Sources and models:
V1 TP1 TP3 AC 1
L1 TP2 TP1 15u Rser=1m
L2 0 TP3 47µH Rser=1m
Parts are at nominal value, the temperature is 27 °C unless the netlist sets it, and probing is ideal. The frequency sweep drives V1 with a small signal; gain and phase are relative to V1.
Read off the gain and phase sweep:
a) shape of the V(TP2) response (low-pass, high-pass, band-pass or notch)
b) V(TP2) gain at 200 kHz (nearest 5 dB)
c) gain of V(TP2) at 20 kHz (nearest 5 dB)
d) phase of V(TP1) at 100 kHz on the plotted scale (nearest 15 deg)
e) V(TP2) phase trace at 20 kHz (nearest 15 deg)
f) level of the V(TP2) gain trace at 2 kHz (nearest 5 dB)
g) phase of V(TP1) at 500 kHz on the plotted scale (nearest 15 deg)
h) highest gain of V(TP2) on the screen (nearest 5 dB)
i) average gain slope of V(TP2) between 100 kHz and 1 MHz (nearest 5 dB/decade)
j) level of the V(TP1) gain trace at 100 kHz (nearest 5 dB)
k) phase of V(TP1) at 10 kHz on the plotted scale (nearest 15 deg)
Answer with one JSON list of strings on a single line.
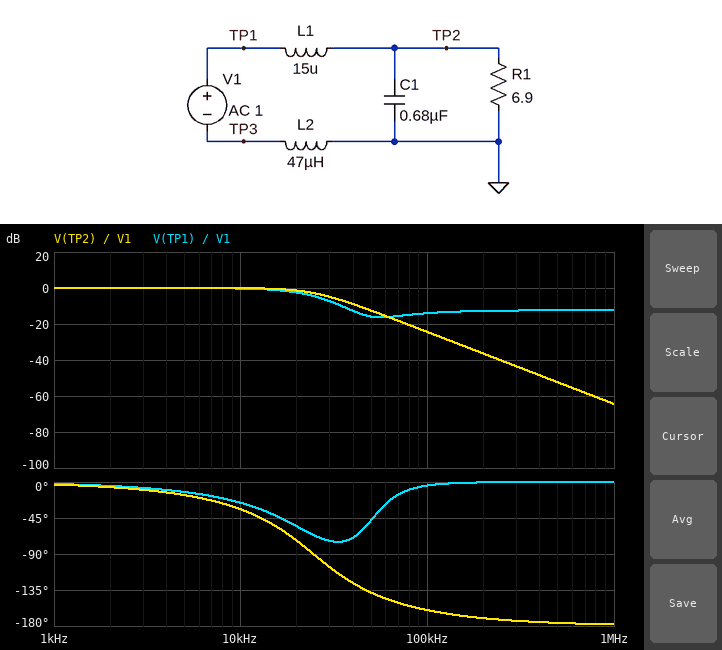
["low-pass", "-35 dB", "0 dB", "0 deg", "-75 deg", "0 dB", "0 deg", "0 dB", "-40 dB/decade", "-15 dB", "-30 deg"]
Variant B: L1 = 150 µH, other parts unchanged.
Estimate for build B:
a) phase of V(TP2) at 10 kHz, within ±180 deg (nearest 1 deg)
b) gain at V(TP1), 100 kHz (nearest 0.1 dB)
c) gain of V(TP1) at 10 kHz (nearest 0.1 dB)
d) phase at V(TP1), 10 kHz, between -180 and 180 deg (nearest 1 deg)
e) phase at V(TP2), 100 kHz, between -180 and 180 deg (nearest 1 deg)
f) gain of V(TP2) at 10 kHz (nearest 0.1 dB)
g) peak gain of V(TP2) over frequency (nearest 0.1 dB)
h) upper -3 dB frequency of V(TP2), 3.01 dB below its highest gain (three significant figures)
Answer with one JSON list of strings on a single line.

["-75 deg", "-2.4 dB", "-1.9 dB", "-9 deg", "-161 deg", "-5.4 dB", "0 dB", "6.62 kHz"]
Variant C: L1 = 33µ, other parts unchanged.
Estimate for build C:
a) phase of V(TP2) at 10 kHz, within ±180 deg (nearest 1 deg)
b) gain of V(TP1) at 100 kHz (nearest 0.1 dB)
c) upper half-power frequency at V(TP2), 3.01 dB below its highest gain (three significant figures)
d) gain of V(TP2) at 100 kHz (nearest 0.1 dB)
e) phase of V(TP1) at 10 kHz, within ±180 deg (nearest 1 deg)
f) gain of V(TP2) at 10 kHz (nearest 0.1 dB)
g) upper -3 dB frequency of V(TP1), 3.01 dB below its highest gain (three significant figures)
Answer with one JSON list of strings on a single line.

["-43 deg", "-8.2 dB", "19.2 kHz", "-26.7 dB", "-25 deg", "-0.6 dB", "16.7 kHz"]
